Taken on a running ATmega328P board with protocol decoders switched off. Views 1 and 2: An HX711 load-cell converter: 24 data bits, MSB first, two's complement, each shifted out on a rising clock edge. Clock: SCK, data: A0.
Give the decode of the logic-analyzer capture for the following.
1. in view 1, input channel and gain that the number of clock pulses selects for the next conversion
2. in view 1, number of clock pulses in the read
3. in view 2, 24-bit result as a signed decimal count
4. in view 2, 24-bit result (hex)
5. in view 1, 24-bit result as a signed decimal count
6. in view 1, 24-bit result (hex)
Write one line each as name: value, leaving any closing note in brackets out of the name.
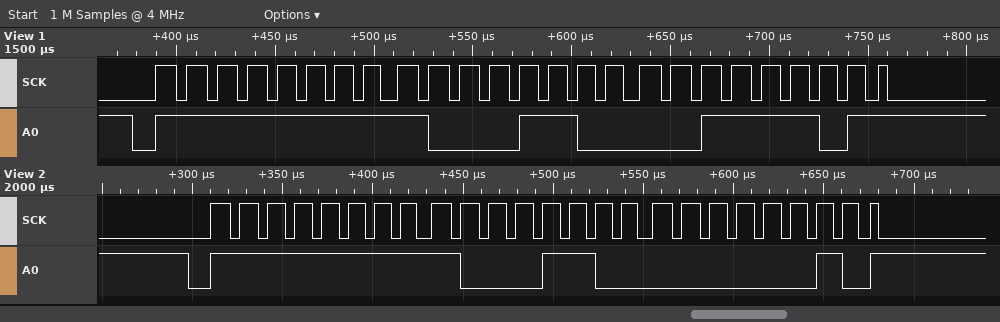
in view 1, input channel and gain that the number of clock pulses selects for the next conversion: channel A, gain 128
in view 1, number of clock pulses in the read: 25
in view 2, 24-bit result as a signed decimal count: -29694
in view 2, 24-bit result: 0xFF8C02
in view 1, 24-bit result as a signed decimal count: -29635
in view 1, 24-bit result: 0xFF8C3D
